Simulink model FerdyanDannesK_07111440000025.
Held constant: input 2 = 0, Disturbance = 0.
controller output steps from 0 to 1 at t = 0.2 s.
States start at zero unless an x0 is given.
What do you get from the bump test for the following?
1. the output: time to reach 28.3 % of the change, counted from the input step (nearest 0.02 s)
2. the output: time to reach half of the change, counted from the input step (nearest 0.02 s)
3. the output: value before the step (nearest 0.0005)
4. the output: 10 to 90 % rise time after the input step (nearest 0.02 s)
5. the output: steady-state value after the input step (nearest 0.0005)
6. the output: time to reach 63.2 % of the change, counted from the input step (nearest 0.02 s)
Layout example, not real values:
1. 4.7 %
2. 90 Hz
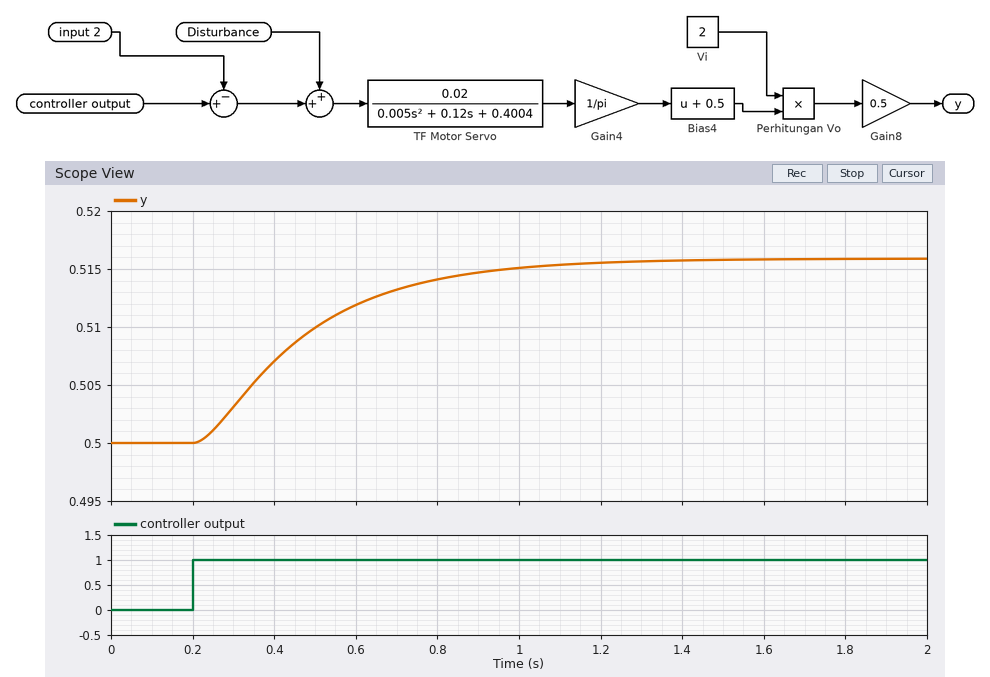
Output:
1. 0.14 s
2. 0.22 s
3. 0.5000
4. 0.56 s
5. 0.5160
6. 0.30 s
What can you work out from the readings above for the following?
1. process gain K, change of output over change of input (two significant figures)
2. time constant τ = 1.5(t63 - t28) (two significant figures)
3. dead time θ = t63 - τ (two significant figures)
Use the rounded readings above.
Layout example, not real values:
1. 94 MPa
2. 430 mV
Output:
1. 0.016
2. 0.24 s
3. 0.060 s
